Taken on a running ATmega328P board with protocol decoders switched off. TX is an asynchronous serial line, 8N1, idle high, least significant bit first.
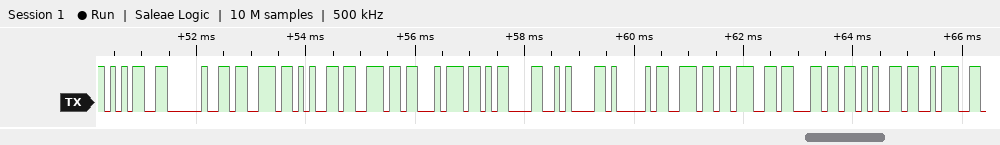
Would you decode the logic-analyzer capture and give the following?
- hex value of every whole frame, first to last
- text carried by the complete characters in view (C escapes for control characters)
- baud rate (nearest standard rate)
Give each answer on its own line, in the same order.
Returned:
0x35 0x20 0x73 0x65 0x6E 0x74 0x0D 0x0A 0x41 0x6E 0x67 0x6C 0x65 0x3A
"5 sent\r\nAngle:"
9600 baud
